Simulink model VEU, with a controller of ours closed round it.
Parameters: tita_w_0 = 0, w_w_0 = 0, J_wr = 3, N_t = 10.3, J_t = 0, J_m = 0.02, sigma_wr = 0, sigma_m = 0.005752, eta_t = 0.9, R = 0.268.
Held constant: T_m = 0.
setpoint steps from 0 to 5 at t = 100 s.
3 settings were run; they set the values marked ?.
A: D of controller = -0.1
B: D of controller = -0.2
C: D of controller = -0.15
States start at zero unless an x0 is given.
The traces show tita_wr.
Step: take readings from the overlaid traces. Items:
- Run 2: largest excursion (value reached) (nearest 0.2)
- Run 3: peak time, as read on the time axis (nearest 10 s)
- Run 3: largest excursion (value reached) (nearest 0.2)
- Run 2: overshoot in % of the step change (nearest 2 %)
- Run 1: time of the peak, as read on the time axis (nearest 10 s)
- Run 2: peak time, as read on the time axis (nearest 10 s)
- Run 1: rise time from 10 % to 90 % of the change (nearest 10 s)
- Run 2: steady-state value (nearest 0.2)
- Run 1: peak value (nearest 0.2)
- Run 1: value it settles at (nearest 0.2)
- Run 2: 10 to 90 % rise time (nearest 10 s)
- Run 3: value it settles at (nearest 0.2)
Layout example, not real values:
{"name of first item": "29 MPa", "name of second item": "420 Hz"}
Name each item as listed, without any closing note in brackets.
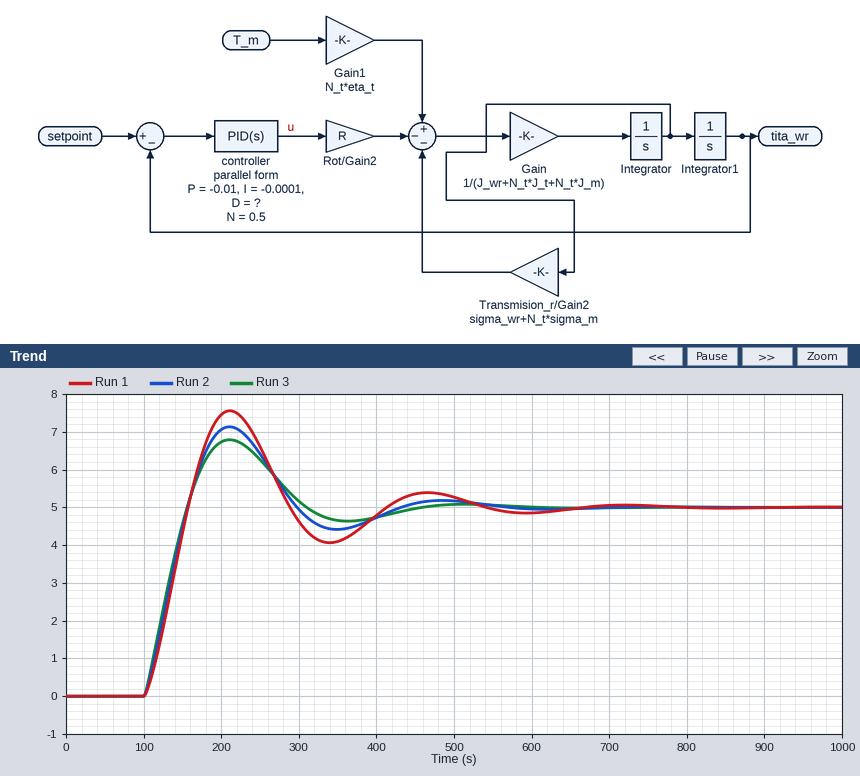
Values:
{"Run 2: largest excursion (value reached)": "7.2", "Run 3: peak time, as read on the time axis": "210 s", "Run 3: largest excursion (value reached)": "6.8", "Run 2: overshoot in % of the step change": "42 %", "Run 1: time of the peak, as read on the time axis": "210 s", "Run 2: peak time, as read on the time axis": "210 s", "Run 1: rise time from 10 % to 90 % of the change": "40 s", "Run 2: steady-state value": "5.0", "Run 1: peak value": "7.6", "Run 1: value it settles at": "5.0", "Run 2: 10 to 90 % rise time": "40 s", "Run 3: value it settles at": "5.0"}
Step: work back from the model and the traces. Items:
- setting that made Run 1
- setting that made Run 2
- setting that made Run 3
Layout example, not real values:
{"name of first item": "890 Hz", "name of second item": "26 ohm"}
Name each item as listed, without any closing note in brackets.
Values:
{"setting that made Run 1": "A", "setting that made Run 2": "C", "setting that made Run 3": "B"}
